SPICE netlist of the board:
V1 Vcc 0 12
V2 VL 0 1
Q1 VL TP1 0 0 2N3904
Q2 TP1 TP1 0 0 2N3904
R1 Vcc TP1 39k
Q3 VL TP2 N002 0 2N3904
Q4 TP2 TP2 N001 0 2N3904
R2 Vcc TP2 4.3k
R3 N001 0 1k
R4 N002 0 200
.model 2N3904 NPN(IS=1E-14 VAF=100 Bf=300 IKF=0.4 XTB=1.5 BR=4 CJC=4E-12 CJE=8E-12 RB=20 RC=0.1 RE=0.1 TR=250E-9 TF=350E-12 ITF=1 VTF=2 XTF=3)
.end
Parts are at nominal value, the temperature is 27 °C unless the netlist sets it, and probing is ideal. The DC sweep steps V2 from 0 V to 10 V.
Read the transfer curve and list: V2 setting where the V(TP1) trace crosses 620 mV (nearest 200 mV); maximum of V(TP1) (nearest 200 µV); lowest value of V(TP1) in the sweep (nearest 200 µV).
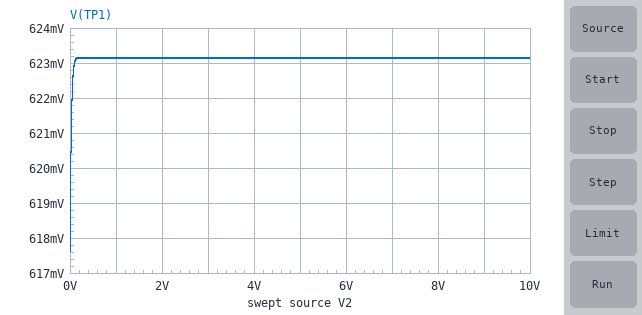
0 V
623.2 mV
617.6 mV
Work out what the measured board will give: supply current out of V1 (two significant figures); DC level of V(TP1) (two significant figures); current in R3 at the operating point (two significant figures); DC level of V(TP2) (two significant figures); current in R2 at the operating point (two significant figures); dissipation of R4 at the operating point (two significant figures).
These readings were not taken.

2.7 mA
620 mV
1.1 mA
1.7 V
2.4 mA
4.8 mW
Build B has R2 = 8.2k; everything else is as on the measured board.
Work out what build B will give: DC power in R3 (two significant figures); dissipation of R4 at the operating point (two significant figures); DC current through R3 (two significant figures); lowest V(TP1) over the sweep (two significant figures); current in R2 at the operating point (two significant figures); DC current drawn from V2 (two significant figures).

1.0 mW
4.5 mW
1.0 mA
620 mV
1.3 mA
4.8 mA
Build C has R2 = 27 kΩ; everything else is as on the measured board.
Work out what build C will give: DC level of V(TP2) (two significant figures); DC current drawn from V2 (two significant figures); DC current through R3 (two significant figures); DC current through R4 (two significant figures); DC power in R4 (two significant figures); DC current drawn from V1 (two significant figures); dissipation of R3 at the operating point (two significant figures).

1.0 V
2.1 mA
400 µA
1.8 mA
650 µW
700 µA
160 µW
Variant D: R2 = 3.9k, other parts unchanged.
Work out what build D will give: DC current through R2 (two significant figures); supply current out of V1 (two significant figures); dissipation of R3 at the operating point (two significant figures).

2.6 mA
2.9 mA
1.2 mW
